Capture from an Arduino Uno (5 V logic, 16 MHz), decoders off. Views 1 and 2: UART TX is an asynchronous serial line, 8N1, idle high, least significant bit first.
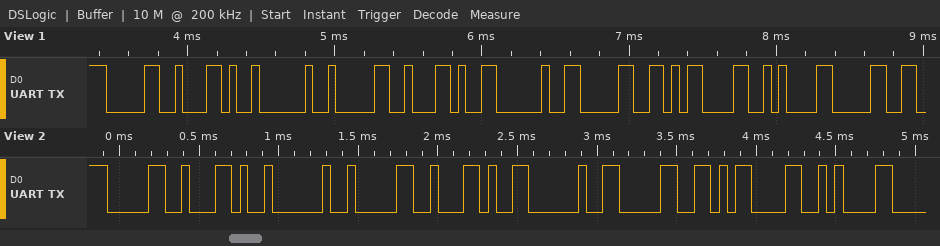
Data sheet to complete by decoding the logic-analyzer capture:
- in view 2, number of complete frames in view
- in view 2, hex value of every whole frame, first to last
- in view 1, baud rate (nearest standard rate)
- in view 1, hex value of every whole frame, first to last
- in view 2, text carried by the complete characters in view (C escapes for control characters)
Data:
9
30 2C 20 30 2C 20 30 0D 0A
19200 baud
0x30 0x2C 0x20 0x30 0x2C 0x20 0x30 0x0D 0x0A 0x30
"0, 0, 0\r\n"
